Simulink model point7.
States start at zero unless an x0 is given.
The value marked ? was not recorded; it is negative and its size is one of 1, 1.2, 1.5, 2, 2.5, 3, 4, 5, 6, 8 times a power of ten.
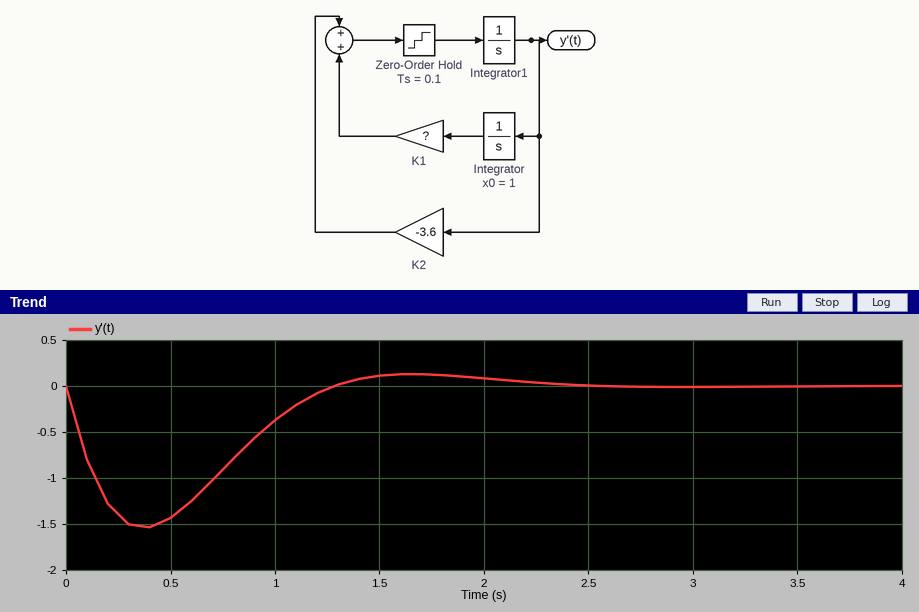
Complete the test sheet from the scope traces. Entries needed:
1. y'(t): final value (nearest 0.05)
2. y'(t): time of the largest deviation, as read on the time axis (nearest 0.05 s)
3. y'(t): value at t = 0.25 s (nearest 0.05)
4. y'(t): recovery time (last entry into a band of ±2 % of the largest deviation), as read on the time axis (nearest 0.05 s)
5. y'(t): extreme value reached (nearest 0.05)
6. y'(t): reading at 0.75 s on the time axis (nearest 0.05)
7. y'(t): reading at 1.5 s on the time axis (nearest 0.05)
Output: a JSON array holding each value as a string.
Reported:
["0.00", "0.40 s", "-1.40", "2.30 s", "-1.55", "-0.90", "0.10"]
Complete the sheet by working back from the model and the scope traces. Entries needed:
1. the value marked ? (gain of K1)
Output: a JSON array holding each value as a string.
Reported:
["-8"]
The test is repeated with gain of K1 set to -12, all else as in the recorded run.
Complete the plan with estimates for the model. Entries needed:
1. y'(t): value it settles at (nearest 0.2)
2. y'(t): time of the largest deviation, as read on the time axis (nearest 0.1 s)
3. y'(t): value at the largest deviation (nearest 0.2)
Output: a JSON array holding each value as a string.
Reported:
["0.0", "0.3 s", "-2.2"]
